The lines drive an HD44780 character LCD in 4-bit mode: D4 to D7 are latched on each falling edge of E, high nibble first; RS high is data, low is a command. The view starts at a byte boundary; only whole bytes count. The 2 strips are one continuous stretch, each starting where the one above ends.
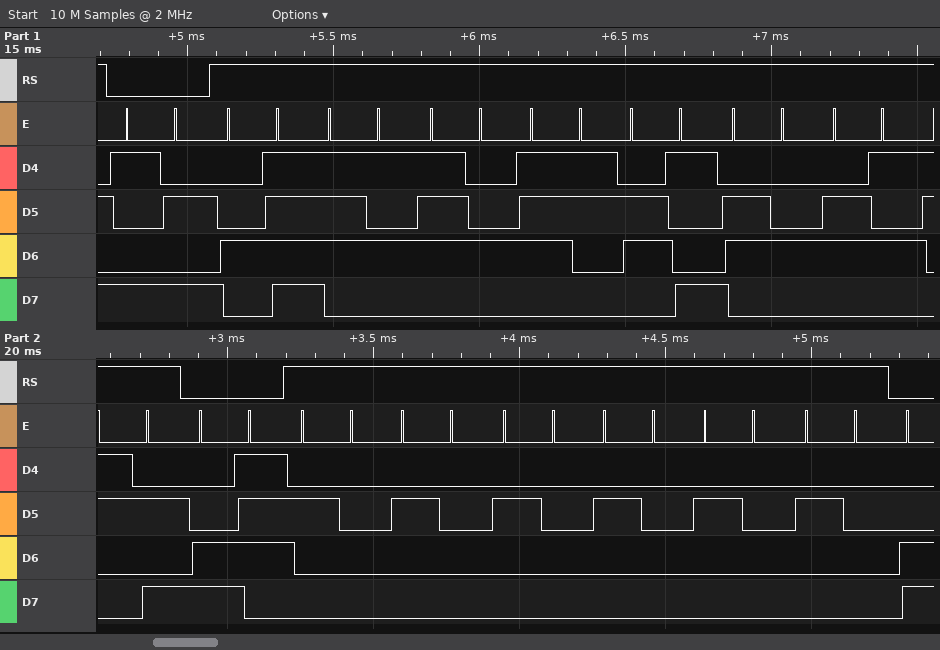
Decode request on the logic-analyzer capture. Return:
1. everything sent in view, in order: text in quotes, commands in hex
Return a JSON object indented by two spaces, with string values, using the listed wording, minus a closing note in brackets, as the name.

{
  "everything sent in view, in order: text in quotes, commands in hex": "0x9A \"Outside:\" 0xC7 \"      \""
}
